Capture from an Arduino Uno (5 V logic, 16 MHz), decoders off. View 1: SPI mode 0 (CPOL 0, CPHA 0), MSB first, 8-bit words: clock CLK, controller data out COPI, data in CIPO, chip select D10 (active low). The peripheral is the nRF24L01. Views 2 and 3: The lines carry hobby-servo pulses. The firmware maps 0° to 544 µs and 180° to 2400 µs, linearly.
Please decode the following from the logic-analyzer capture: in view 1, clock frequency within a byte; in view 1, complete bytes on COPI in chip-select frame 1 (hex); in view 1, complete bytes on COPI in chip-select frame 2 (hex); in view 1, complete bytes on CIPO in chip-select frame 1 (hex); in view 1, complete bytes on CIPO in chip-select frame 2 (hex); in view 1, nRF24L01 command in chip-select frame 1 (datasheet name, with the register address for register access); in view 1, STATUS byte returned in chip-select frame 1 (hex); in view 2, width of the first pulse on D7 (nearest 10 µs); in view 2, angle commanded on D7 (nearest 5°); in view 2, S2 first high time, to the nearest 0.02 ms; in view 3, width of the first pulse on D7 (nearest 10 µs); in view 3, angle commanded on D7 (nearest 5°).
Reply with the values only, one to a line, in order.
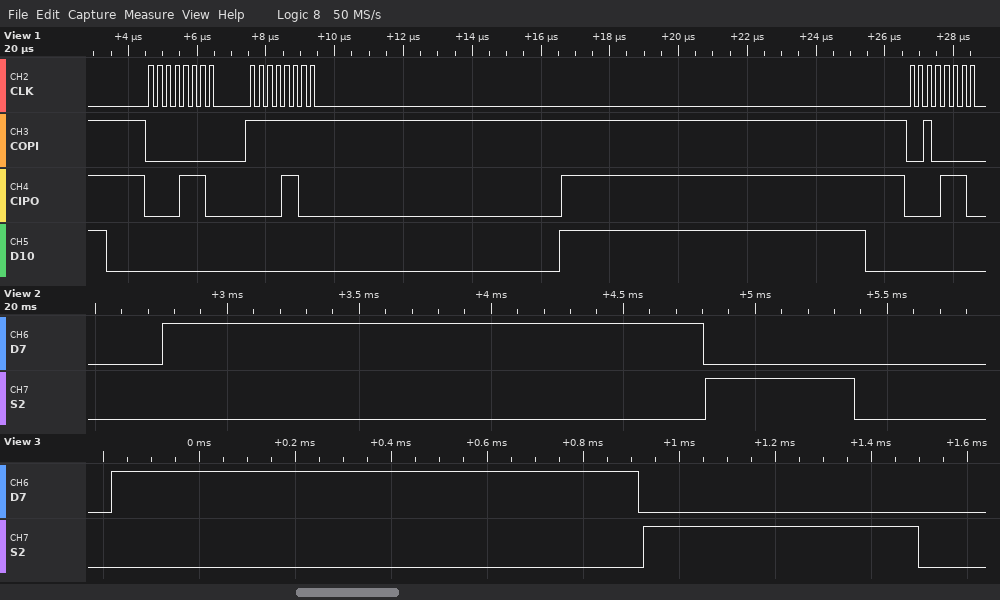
4 MHz
00 FF
20
0E 0C
0E
R_REGISTER 0x00
0x0E
2050 µs
145°
0.56 ms
1100 µs
55°
